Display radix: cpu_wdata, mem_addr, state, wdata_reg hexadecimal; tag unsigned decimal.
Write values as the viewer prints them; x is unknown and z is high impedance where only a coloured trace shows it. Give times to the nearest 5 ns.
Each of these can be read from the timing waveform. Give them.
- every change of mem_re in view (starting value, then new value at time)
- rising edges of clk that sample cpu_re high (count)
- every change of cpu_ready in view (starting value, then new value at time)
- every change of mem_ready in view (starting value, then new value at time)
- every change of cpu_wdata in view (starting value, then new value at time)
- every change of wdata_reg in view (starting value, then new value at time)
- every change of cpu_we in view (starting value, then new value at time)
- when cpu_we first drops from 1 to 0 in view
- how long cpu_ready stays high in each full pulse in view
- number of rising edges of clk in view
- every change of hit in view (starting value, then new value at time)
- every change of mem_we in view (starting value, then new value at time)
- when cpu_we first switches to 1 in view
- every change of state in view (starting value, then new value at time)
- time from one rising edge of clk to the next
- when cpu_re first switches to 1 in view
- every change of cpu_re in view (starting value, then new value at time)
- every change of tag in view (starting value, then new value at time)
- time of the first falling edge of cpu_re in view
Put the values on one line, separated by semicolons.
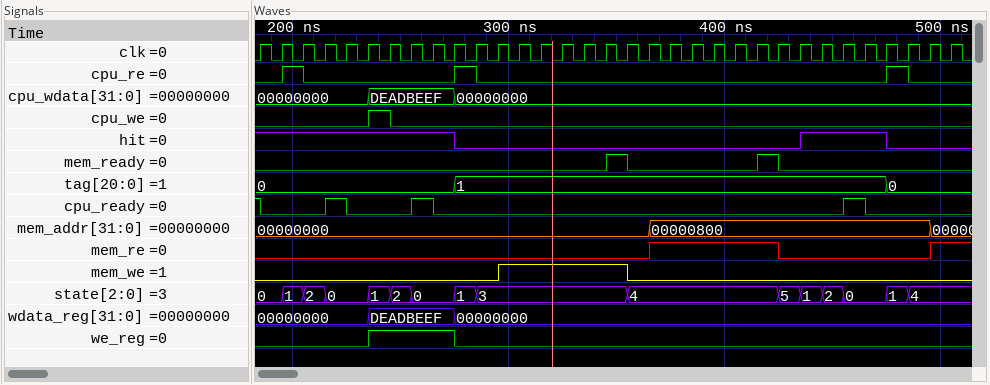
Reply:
0, 1 at 365 ns, 0 at 425 ns, 1 at 495 ns; 3; 1, 0 at 185 ns, 1 at 215 ns, 0 at 225 ns, 1 at 255 ns, 0 at 265 ns, 1 at 455 ns, 0 at 465 ns; 0, 1 at 345 ns, 0 at 355 ns, 1 at 415 ns, 0 at 425 ns; 00000000, DEADBEEF at 235 ns, 00000000 at 275 ns; 00000000, DEADBEEF at 235 ns, 00000000 at 275 ns; 0, 1 at 235 ns, 0 at 245 ns; 245 ns; 10 ns, 10 ns, 10 ns; 33; 1, 0 at 275 ns, 1 at 435 ns, 0 at 475 ns; 0, 1 at 295 ns, 0 at 355 ns; 235 ns; 0, 1 at 195 ns, 2 at 205 ns, 0 at 215 ns, 1 at 235 ns, 2 at 245 ns, 0 at 255 ns, 1 at 275 ns, 3 at 285 ns, 4 at 355 ns, 5 at 425 ns, 1 at 435 ns, 2 at 445 ns, 0 at 455 ns, 1 at 475 ns, 4 at 485 ns; 10 ns; 195 ns; 0, 1 at 195 ns, 0 at 205 ns, 1 at 275 ns, 0 at 285 ns, 1 at 475 ns, 0 at 485 ns; 0, 1 at 275 ns, 0 at 475 ns; 205 ns
